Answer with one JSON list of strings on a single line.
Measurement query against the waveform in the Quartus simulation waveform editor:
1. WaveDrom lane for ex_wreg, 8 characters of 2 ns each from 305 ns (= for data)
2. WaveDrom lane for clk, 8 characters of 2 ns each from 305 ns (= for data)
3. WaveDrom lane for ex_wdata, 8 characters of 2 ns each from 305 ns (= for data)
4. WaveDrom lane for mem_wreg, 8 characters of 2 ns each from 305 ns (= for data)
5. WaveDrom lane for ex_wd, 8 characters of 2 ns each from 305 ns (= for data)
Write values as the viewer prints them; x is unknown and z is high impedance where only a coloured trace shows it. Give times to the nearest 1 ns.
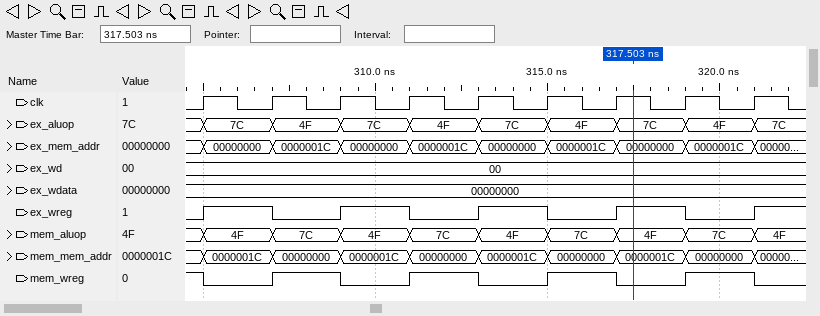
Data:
["{name: 'ex_wreg', wave: '10101010'}", "{name: 'clk', wave: 'p.......'}", "{name: 'ex_wdata', wave: '=.......', data: '00000000'}", "{name: 'mem_wreg', wave: '01010101'}", "{name: 'ex_wd', wave: '=.......', data: '00'}"]
